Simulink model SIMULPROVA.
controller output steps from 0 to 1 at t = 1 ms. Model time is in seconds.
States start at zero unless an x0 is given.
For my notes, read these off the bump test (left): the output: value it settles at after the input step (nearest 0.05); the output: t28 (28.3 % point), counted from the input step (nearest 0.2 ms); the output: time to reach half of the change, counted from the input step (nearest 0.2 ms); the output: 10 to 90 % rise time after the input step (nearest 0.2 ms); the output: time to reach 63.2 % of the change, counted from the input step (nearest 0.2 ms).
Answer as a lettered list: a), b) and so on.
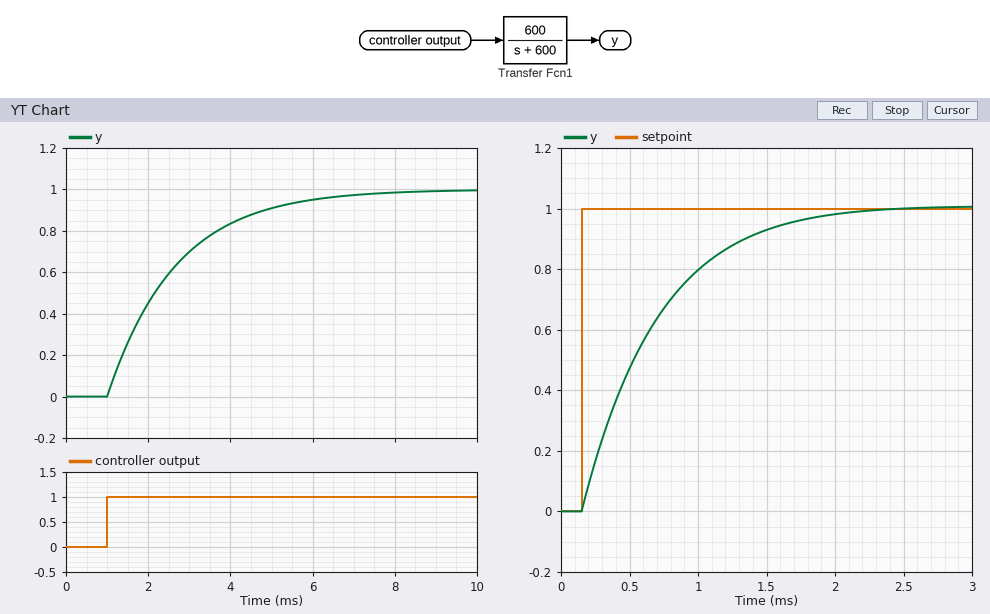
a) 1.00
b) 0.6 ms
c) 1.2 ms
d) 3.6 ms
e) 1.6 ms
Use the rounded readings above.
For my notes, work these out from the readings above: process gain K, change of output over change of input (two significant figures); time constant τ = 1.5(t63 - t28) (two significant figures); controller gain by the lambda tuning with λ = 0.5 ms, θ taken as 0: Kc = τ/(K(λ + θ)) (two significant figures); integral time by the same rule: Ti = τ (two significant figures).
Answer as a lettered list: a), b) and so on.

a) 1.0
b) 1.5 ms
c) 3.0
d) 1.5 ms
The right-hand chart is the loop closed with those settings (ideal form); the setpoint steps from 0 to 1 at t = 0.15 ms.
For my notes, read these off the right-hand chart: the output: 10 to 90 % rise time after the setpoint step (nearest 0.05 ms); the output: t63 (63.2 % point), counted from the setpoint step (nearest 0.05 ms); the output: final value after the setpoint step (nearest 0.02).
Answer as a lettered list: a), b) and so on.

a) 1.15 ms
b) 0.55 ms
c) 1.00
